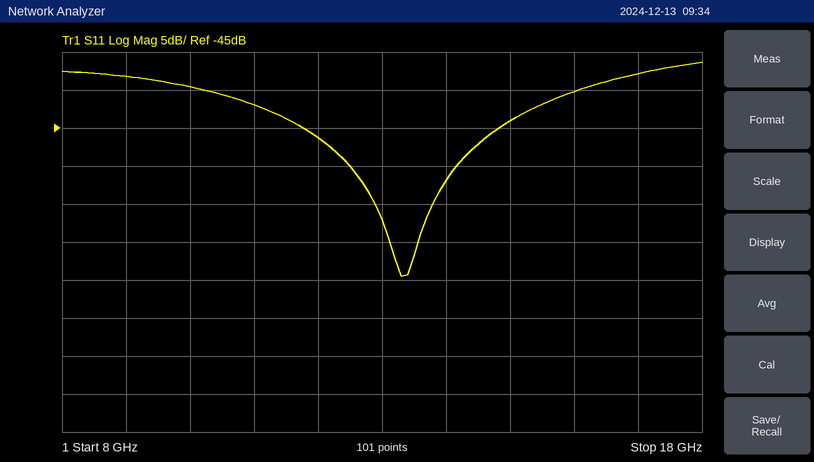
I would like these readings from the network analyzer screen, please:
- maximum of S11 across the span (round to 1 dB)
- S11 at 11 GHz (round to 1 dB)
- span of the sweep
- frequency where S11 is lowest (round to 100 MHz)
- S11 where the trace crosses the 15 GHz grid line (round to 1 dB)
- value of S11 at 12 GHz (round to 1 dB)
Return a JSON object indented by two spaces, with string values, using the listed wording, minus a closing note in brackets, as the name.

{
  "maximum of S11 across the span": "-36 dB",
  "S11 at 11 GHz": "-42 dB",
  "span of the sweep": "10 GHz",
  "frequency where S11 is lowest": "13.3 GHz",
  "S11 where the trace crosses the 15 GHz grid line": "-44 dB",
  "value of S11 at 12 GHz": "-46 dB"
}
